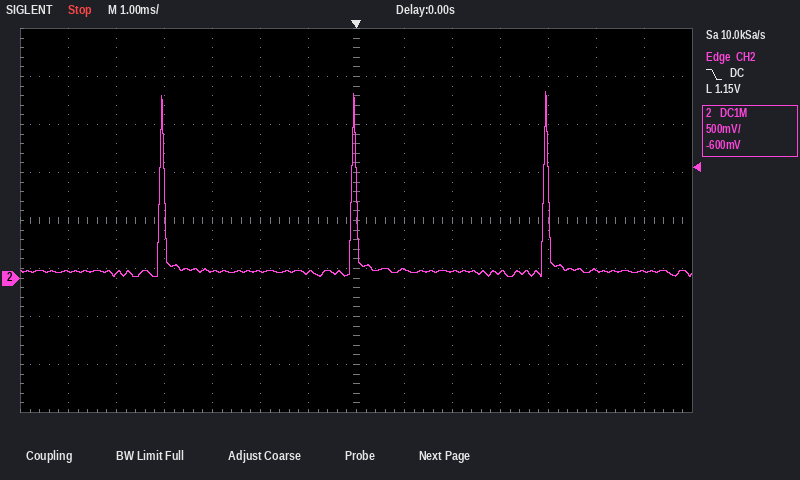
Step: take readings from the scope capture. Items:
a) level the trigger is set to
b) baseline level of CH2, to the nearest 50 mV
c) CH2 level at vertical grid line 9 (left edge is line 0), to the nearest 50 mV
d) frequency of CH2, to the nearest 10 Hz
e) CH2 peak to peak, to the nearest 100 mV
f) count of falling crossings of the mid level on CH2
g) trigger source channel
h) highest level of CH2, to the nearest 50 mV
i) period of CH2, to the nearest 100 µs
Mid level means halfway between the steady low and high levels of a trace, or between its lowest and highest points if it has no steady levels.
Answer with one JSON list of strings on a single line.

["1.15 V", "50 mV", "50 mV", "250 Hz", "1.90 V", "3", "CH2", "1.95 V", "4.0 ms"]
